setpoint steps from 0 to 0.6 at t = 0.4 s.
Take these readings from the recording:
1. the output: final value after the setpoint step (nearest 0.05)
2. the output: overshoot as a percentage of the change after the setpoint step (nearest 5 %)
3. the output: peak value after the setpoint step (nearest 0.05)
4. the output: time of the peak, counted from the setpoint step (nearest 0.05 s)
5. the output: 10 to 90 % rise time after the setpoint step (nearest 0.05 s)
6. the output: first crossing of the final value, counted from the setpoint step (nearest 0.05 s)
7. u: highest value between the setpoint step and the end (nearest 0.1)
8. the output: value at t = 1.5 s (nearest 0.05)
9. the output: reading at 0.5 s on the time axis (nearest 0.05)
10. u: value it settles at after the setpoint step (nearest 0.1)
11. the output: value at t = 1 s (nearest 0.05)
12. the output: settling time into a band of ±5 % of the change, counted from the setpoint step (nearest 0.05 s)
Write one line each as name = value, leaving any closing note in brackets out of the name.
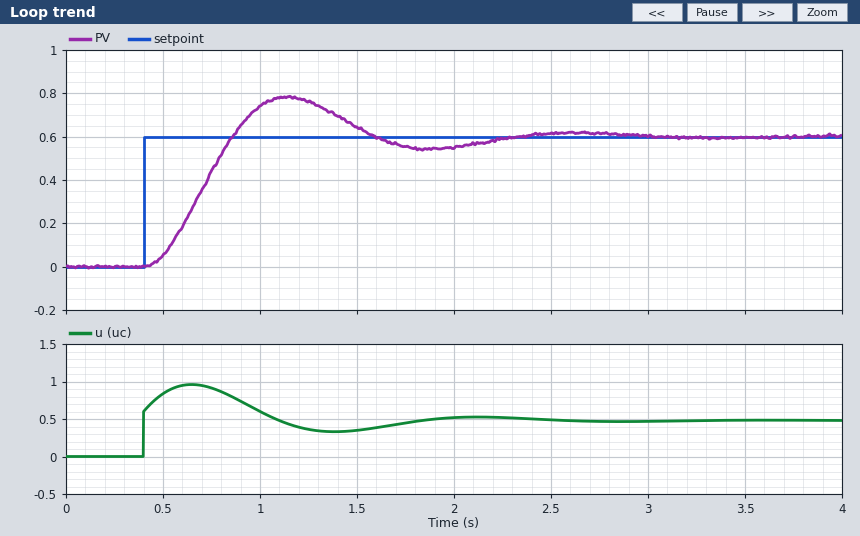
the output: final value after the setpoint step = 0.60
the output: overshoot as a percentage of the change after the setpoint step = 30 %
the output: peak value after the setpoint step = 0.80
the output: time of the peak, counted from the setpoint step = 0.75 s
the output: 10 to 90 % rise time after the setpoint step = 0.30 s
the output: first crossing of the final value, counted from the setpoint step = 0.45 s
u: highest value between the setpoint step and the end = 1.0
the output: value at t = 1.5 s = 0.65
the output: reading at 0.5 s on the time axis = 0.05
u: value it settles at after the setpoint step = 0.5
the output: value at t = 1 s = 0.75
the output: settling time into a band of ±5 % of the change, counted from the setpoint step = 1.75 s
